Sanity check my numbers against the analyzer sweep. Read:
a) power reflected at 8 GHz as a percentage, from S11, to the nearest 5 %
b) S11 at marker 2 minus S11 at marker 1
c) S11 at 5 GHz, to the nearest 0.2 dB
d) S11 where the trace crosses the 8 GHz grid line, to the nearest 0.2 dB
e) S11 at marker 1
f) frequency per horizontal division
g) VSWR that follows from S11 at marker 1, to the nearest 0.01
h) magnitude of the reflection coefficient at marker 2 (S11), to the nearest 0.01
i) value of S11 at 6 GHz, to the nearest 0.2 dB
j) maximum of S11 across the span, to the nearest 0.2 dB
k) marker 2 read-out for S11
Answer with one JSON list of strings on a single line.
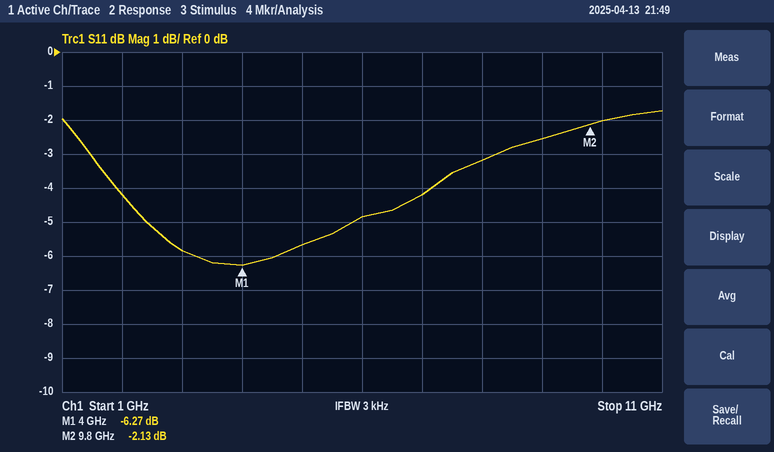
["50 %", "4.14 dB", "-5.6 dB", "-3.2 dB", "-6.27 dB", "1 GHz", "2.89", "0.78", "-4.8 dB", "-1.8 dB", "-2.13 dB"]
